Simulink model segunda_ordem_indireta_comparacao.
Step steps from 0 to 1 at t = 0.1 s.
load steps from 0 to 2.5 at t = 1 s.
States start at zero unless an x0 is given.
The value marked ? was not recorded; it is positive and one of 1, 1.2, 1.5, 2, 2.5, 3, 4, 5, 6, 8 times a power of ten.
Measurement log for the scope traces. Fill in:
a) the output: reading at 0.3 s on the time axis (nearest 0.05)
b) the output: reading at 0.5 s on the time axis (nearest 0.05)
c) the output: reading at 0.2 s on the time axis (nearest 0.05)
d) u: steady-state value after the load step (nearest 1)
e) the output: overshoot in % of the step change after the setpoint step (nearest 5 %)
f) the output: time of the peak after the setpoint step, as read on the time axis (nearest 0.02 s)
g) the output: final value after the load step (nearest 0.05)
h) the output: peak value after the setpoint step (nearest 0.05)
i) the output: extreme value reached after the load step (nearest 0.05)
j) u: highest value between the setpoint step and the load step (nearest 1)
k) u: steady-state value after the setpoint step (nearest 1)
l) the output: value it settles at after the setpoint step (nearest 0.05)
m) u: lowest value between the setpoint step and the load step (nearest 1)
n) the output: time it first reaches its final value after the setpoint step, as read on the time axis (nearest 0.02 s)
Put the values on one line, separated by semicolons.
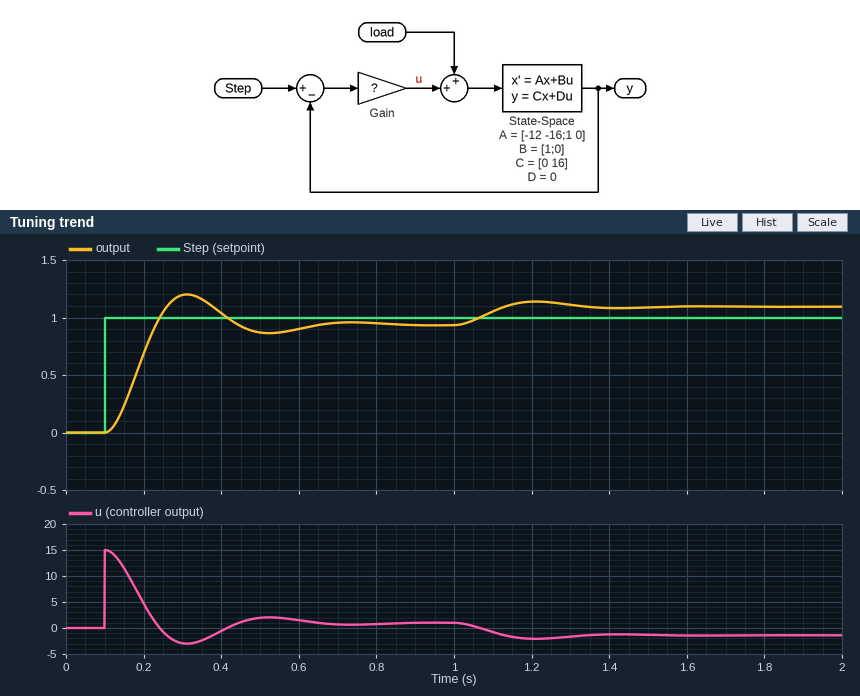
1.20; 0.85; 0.70; -1; 30 %; 0.32 s; 1.10; 1.20; 1.15; 15; 1; 0.95; -3; 0.24 s
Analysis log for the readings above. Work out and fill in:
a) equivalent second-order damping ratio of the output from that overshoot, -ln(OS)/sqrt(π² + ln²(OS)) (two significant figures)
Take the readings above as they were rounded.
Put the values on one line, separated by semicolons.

0.36
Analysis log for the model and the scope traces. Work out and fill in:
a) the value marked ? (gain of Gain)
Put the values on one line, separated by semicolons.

15
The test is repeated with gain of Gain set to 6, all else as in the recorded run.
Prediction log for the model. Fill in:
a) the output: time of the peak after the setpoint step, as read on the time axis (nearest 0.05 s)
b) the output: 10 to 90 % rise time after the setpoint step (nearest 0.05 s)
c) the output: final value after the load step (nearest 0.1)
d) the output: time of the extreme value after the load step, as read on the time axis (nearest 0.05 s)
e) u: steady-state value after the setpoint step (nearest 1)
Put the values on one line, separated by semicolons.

0.45 s; 0.15 s; 1.2; 1.35 s; 1
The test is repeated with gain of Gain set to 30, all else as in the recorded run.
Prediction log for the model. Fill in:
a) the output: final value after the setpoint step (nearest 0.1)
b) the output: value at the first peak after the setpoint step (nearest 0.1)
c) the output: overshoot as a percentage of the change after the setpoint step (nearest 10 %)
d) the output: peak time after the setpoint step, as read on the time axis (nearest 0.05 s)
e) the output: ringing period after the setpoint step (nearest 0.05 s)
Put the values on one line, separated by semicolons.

1.0; 1.4; 40 %; 0.25 s; 0.30 s
